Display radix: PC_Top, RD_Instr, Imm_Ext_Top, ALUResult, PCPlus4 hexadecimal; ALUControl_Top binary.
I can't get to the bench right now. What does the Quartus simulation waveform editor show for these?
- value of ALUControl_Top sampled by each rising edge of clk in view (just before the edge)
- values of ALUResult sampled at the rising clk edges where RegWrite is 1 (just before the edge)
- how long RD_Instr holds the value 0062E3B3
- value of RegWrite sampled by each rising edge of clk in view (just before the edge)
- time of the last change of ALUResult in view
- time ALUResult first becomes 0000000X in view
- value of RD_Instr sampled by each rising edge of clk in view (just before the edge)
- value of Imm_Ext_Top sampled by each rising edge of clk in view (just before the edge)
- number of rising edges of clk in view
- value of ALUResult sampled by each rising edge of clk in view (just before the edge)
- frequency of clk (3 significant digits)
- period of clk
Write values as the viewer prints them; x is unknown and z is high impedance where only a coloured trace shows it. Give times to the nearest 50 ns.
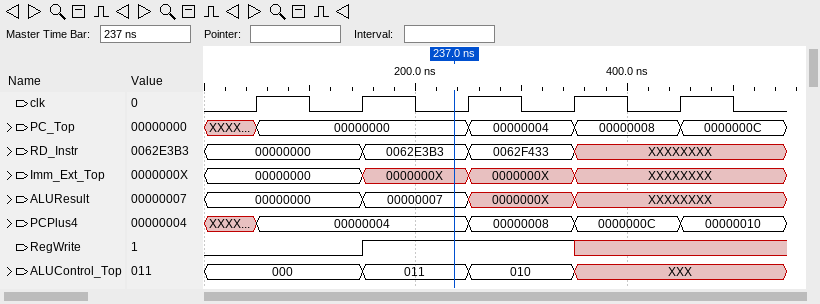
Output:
000, 000, 011, 010, XXX
00000007, 0000000X
100 ns
0 0 1 1 x
350 ns
250 ns
00000000, 00000000, 0062E3B3, 0062F433, XXXXXXXX
00000000, 00000000, 0000000X, 0000000X, XXXXXXXX
5
00000000, 00000000, 00000007, 0000000X, XXXXXXXX
10.0 MHz
100 ns
